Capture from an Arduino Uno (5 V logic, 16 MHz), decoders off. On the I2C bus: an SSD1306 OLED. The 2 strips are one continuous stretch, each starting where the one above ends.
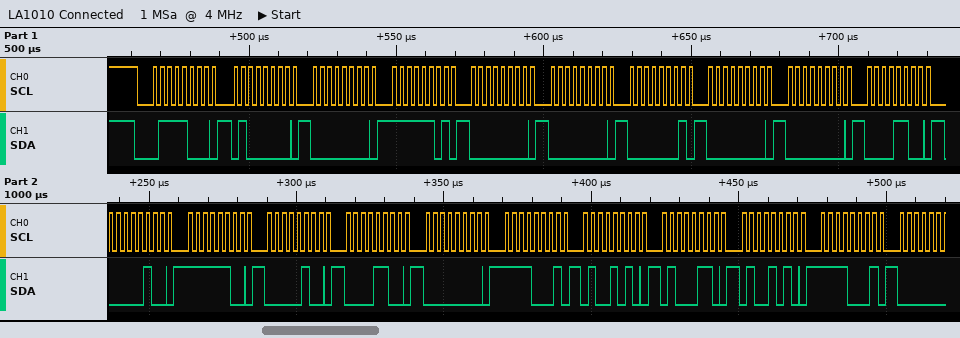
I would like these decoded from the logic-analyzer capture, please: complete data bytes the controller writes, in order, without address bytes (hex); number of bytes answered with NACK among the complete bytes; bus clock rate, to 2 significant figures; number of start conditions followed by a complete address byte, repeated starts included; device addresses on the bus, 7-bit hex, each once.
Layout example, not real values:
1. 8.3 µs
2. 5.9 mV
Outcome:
1. 40 00 FD 00 00 01 00 00 0C 04 FC 04 0C 00 F1 4A 46 4A F1
2. 0
3. 400 kHz
4. 1
5. 0x3C
